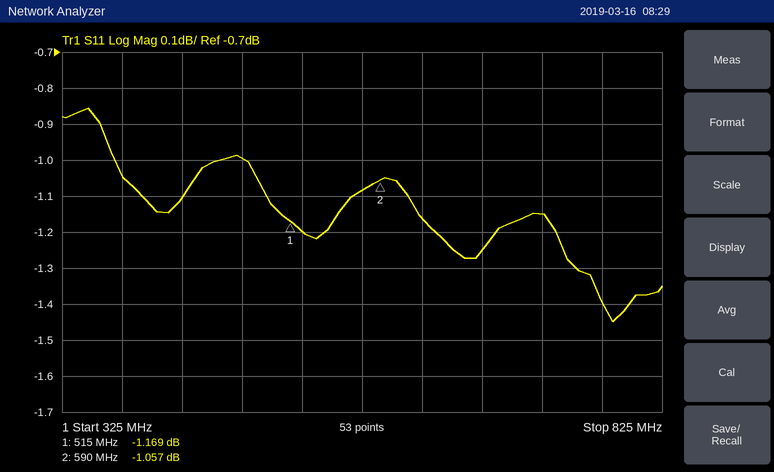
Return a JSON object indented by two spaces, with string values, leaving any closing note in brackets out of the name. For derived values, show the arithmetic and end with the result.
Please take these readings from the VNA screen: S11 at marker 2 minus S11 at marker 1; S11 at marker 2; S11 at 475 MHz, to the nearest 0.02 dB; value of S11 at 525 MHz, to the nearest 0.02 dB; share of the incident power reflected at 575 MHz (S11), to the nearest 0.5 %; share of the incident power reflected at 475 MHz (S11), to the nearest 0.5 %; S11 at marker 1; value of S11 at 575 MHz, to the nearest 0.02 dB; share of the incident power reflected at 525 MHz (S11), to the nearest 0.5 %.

{
  "S11 at marker 2 minus S11 at marker 1": "-1.057 − (-1.169) = 0.112 dB",
  "S11 at marker 2": "-1.057 dB",
  "S11 at 475 MHz, to the nearest 0.02 dB": "-1.00 dB",
  "value of S11 at 525 MHz, to the nearest 0.02 dB": "-1.20 dB",
  "share of the incident power reflected at 575 MHz (S11), to the nearest 0.5 %": "10^(-1.08/10) ≈ 78.0 %",
  "share of the incident power reflected at 475 MHz (S11), to the nearest 0.5 %": "10^(-1/10) ≈ 79.4 %, so 79.5 % to the nearest 0.5 %",
  "S11 at marker 1": "-1.169 dB",
  "value of S11 at 575 MHz, to the nearest 0.02 dB": "-1.08 dB",
  "share of the incident power reflected at 525 MHz (S11), to the nearest 0.5 %": "10^(-1.2/10) ≈ 75.9 %, so 76.0 % to the nearest 0.5 %"
}
